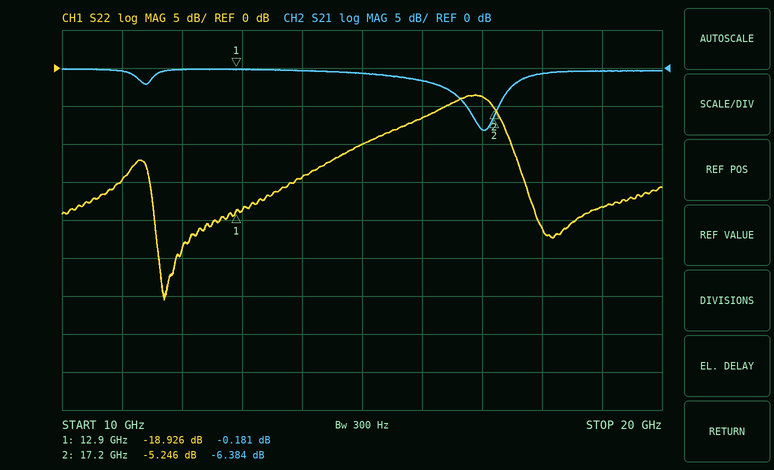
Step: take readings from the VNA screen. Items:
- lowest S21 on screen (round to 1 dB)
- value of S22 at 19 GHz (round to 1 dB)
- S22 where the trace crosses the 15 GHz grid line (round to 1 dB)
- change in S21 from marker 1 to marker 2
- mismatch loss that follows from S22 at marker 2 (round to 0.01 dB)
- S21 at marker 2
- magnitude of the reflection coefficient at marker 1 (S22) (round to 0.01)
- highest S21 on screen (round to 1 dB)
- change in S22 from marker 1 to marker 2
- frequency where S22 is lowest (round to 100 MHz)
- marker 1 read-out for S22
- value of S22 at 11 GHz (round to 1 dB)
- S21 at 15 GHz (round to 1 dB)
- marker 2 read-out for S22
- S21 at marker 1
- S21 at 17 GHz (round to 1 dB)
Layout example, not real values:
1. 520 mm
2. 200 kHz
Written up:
1. -8 dB
2. -18 dB
3. -10 dB
4. -6.203 dB
5. 1.54 dB
6. -6.384 dB
7. 0.11
8. 0 dB
9. 13.680 dB
10. 11.7 GHz
11. -18.926 dB
12. -15 dB
13. -1 dB
14. -5.246 dB
15. -0.181 dB
16. -8 dB
